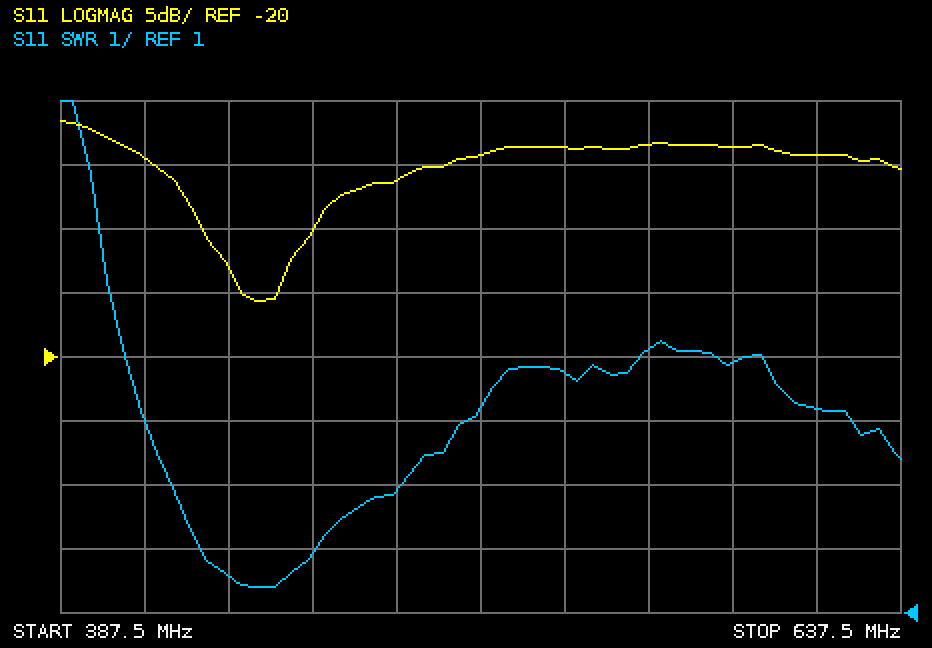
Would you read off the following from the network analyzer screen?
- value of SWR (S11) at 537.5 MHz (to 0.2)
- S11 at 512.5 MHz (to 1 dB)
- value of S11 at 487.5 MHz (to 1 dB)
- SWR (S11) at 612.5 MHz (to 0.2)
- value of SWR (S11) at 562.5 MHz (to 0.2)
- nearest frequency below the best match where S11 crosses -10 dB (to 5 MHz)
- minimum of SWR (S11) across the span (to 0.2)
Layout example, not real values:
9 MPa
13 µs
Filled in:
4.8
-4 dB
-6 dB
4.2
5.2
430 MHz
1.4
